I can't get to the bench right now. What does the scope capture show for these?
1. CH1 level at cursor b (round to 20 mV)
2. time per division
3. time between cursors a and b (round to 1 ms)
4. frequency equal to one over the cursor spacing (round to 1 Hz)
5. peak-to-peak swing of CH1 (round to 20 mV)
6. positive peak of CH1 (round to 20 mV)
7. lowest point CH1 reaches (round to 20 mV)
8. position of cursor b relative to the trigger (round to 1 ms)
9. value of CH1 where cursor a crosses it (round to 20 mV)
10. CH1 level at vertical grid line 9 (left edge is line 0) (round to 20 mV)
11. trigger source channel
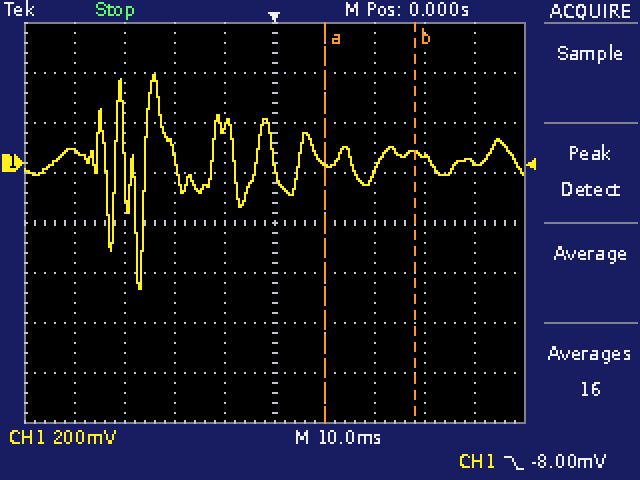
40 mV
10 ms
18 ms
56 Hz
860 mV
360 mV
-500 mV
+28 ms
0 mV
0 mV
CH1
